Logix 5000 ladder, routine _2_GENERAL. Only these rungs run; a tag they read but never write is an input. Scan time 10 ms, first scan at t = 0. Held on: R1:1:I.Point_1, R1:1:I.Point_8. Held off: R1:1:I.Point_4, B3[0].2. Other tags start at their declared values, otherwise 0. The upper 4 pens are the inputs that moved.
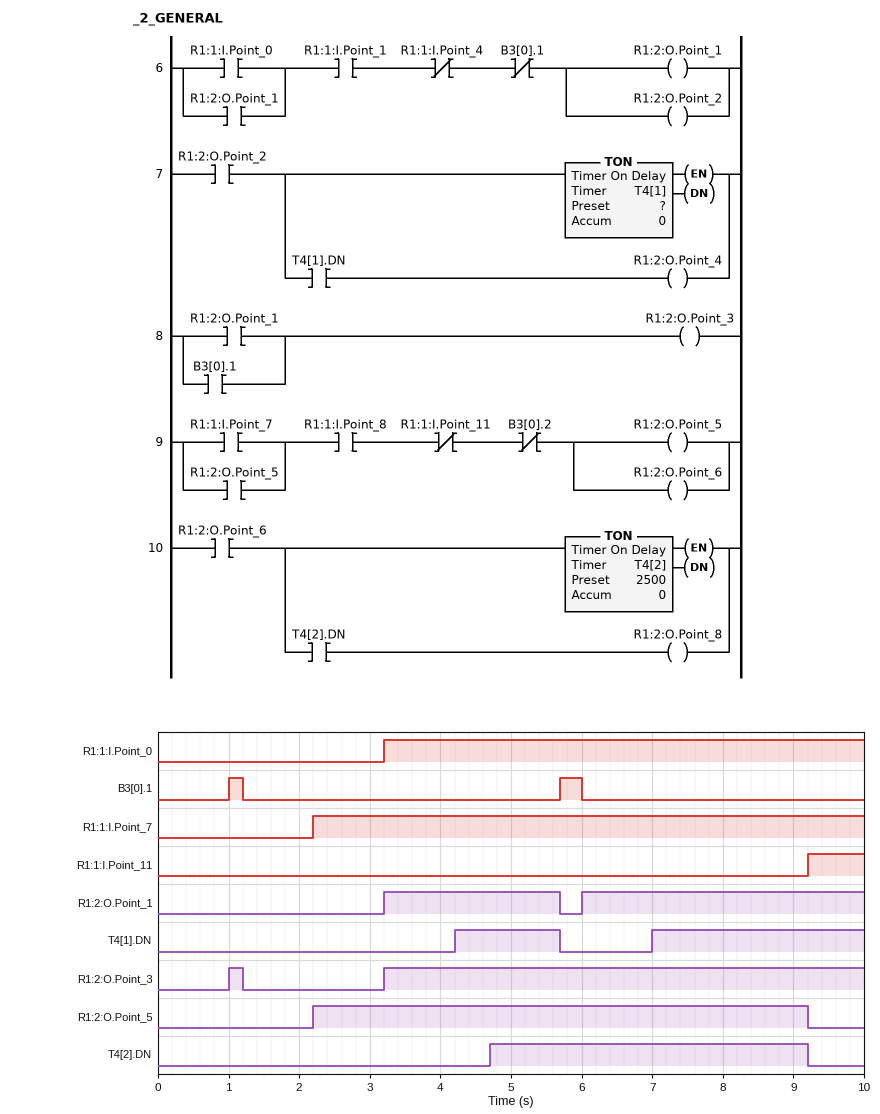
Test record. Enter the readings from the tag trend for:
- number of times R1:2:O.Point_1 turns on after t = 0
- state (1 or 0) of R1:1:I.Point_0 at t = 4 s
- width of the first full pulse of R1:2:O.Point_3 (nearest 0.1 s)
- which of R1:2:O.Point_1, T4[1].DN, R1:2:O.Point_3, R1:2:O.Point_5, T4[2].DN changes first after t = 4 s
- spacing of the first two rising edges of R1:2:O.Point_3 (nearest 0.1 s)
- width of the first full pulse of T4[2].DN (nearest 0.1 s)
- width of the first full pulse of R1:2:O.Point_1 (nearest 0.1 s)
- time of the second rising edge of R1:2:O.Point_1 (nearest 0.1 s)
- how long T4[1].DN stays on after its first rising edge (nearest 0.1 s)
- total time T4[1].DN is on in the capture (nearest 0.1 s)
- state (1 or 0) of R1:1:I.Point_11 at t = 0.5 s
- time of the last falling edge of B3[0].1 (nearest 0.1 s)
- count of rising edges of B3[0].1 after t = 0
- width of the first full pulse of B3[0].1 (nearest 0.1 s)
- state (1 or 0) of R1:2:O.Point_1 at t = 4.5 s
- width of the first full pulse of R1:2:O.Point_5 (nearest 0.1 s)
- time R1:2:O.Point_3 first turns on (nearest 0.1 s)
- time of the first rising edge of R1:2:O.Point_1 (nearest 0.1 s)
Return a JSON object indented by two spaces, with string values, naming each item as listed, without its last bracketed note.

{
  "number of times R1:2:O.Point_1 turns on after t = 0": "2",
  "state (1 or 0) of R1:1:I.Point_0 at t = 4 s": "1",
  "width of the first full pulse of R1:2:O.Point_3": "0.2 s",
  "which of R1:2:O.Point_1, T4[1].DN, R1:2:O.Point_3, R1:2:O.Point_5, T4[2].DN changes first after t = 4 s": "T4[1].DN",
  "spacing of the first two rising edges of R1:2:O.Point_3": "2.2 s",
  "width of the first full pulse of T4[2].DN": "4.5 s",
  "width of the first full pulse of R1:2:O.Point_1": "2.5 s",
  "time of the second rising edge of R1:2:O.Point_1": "6.0 s",
  "how long T4[1].DN stays on after its first rising edge": "1.5 s",
  "total time T4[1].DN is on in the capture": "4.5 s",
  "state (1 or 0) of R1:1:I.Point_11 at t = 0.5 s": "0",
  "time of the last falling edge of B3[0].1": "6.0 s",
  "count of rising edges of B3[0].1 after t = 0": "2",
  "width of the first full pulse of B3[0].1": "0.2 s",
  "state (1 or 0) of R1:2:O.Point_1 at t = 4.5 s": "1",
  "width of the first full pulse of R1:2:O.Point_5": "7.0 s",
  "time R1:2:O.Point_3 first turns on": "1.0 s",
  "time of the first rising edge of R1:2:O.Point_1": "3.2 s"
}
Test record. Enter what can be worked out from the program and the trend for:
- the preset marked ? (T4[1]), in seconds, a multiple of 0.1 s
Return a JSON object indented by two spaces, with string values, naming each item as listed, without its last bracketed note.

{
  "the preset marked ? (T4[1]), in seconds, a multiple of 0.1 s": "1.0 s"
}
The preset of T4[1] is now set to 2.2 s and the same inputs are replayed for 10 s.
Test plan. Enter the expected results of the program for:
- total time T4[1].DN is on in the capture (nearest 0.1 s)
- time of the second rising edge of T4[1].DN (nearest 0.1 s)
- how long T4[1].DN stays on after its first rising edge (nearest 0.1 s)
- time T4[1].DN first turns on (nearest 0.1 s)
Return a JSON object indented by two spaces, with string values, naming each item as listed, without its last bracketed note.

{
  "total time T4[1].DN is on in the capture": "2.1 s",
  "time of the second rising edge of T4[1].DN": "8.2 s",
  "how long T4[1].DN stays on after its first rising edge": "0.3 s",
  "time T4[1].DN first turns on": "5.4 s"
}
